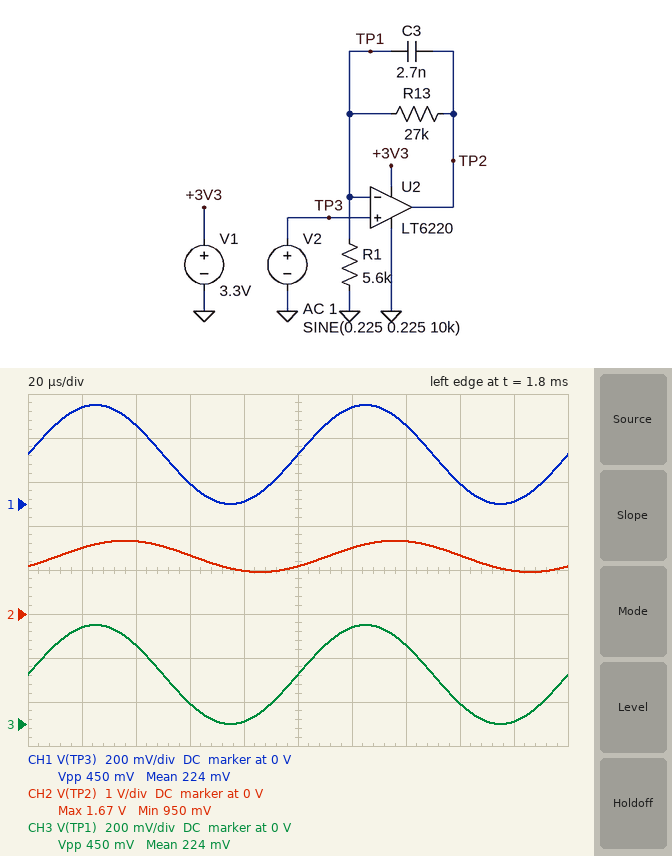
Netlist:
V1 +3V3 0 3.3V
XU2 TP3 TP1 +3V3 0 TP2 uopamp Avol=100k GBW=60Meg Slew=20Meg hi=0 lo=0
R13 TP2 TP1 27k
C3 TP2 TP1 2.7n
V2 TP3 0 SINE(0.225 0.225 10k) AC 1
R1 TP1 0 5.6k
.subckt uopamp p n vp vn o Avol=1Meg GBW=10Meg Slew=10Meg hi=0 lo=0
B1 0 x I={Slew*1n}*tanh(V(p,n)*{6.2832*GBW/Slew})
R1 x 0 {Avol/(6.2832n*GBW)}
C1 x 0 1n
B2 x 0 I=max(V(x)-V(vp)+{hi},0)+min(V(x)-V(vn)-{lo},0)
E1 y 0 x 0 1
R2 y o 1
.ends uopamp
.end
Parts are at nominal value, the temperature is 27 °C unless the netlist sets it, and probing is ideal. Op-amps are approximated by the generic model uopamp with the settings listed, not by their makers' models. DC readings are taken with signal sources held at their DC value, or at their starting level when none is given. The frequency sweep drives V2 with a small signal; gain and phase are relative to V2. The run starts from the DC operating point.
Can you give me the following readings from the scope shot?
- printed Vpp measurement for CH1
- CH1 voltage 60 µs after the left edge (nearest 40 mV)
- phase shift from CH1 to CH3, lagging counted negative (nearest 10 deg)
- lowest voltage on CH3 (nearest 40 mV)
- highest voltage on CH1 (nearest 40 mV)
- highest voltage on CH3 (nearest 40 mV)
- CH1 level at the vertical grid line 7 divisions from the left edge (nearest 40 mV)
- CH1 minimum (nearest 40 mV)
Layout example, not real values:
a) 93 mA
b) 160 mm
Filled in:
a) 450 mV
b) 80 mV
c) 0 deg
d) 0 V
e) 440 mV
f) 440 mV
g) 360 mV
h) 0 V
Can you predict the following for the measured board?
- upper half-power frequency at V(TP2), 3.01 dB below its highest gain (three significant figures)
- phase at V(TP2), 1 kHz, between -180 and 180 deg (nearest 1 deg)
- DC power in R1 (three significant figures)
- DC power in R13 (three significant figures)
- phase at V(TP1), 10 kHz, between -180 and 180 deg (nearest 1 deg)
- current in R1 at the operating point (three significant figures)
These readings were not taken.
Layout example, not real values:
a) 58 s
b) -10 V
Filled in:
a) 2.25 kHz
b) -20 deg
c) 9.04 µW
d) 43.6 µW
e) 0 deg
f) 40.2 µA
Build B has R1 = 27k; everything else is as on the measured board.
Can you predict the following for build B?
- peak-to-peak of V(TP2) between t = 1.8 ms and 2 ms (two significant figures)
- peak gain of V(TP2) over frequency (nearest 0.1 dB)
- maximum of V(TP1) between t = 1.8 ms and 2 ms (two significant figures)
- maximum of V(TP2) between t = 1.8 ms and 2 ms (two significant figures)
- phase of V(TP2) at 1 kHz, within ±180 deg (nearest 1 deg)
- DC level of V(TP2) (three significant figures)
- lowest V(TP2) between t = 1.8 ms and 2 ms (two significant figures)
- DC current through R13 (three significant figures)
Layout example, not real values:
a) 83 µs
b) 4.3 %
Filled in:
a) 480 mV
b) 6.0 dB
c) 450 mV
d) 690 mV
e) -12 deg
f) 450 mV
g) 210 mV
h) 8.33 µA
